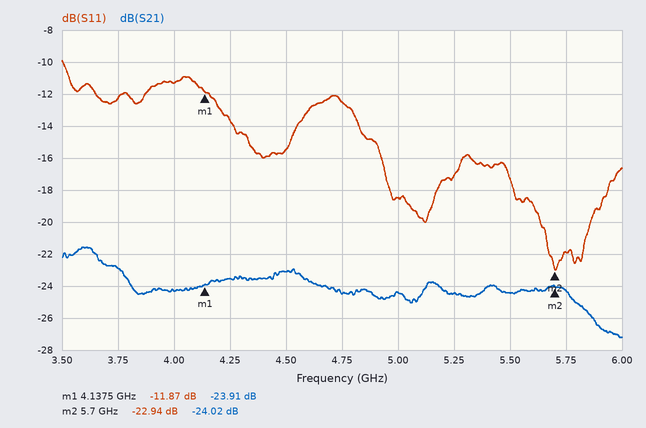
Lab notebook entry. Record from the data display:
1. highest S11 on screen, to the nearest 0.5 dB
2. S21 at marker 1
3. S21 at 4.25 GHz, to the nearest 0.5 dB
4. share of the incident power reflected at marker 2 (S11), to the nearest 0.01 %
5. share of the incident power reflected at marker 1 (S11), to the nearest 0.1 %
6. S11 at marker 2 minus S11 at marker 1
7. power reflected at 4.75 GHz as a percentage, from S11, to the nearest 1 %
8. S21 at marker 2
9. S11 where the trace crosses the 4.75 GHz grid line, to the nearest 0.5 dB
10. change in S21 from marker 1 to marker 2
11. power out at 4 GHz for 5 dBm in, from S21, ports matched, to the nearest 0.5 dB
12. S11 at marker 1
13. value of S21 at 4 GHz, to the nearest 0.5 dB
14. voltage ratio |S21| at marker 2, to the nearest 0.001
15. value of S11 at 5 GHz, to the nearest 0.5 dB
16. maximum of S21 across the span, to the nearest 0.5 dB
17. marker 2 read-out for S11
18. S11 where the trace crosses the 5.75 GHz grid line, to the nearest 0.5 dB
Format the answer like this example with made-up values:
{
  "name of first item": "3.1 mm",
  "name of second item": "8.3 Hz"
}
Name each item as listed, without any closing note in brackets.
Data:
{
  "highest S11 on screen, to the nearest 0.5 dB": "-10.0 dB",
  "S21 at marker 1": "-23.91 dB",
  "S21 at 4.25 GHz, to the nearest 0.5 dB": "-23.5 dB",
  "share of the incident power reflected at marker 2 (S11), to the nearest 0.01 %": "0.51 %",
  "share of the incident power reflected at marker 1 (S11), to the nearest 0.1 %": "6.5 %",
  "S11 at marker 2 minus S11 at marker 1": "-11.07 dB",
  "power reflected at 4.75 GHz as a percentage, from S11, to the nearest 1 %": "6 %",
  "S21 at marker 2": "-24.02 dB",
  "S11 where the trace crosses the 4.75 GHz grid line, to the nearest 0.5 dB": "-12.5 dB",
  "change in S21 from marker 1 to marker 2": "-0.11 dB",
  "power out at 4 GHz for 5 dBm in, from S21, ports matched, to the nearest 0.5 dB": "-19.5 dBm",
  "S11 at marker 1": "-11.87 dB",
  "value of S21 at 4 GHz, to the nearest 0.5 dB": "-24.5 dB",
  "voltage ratio |S21| at marker 2, to the nearest 0.001": "0.063",
  "value of S11 at 5 GHz, to the nearest 0.5 dB": "-18.5 dB",
  "maximum of S21 across the span, to the nearest 0.5 dB": "-21.5 dB",
  "marker 2 read-out for S11": "-22.94 dB",
  "S11 where the trace crosses the 5.75 GHz grid line, to the nearest 0.5 dB": "-22.0 dB"
}
